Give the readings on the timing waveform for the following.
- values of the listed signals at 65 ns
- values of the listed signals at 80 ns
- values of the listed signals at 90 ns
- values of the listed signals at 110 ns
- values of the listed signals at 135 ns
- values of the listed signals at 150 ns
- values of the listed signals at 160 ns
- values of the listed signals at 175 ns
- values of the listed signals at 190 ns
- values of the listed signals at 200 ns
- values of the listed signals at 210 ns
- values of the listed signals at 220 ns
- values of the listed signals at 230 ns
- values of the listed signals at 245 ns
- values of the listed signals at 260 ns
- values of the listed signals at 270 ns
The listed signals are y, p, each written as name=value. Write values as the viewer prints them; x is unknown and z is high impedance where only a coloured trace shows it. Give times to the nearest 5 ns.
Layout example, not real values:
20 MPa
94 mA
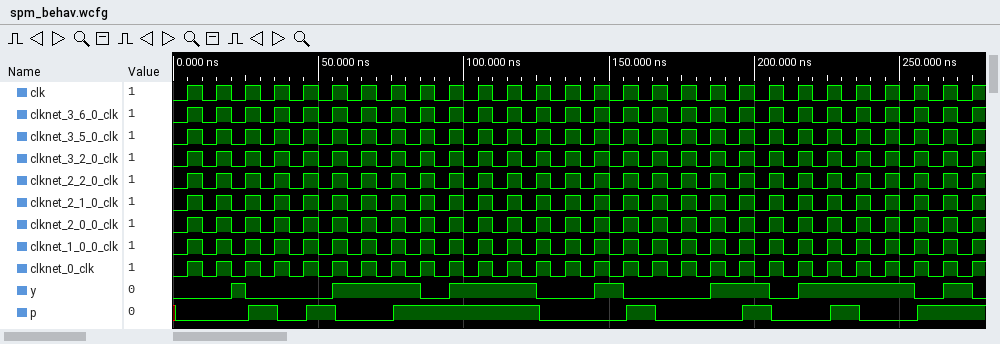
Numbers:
y=1, p=0
y=1, p=1
y=0, p=1
y=1, p=1
y=0, p=0
y=1, p=0
y=0, p=1
y=0, p=0
y=1, p=0
y=1, p=1
y=0, p=0
y=1, p=0
y=1, p=1
y=1, p=0
y=0, p=1
y=1, p=1
